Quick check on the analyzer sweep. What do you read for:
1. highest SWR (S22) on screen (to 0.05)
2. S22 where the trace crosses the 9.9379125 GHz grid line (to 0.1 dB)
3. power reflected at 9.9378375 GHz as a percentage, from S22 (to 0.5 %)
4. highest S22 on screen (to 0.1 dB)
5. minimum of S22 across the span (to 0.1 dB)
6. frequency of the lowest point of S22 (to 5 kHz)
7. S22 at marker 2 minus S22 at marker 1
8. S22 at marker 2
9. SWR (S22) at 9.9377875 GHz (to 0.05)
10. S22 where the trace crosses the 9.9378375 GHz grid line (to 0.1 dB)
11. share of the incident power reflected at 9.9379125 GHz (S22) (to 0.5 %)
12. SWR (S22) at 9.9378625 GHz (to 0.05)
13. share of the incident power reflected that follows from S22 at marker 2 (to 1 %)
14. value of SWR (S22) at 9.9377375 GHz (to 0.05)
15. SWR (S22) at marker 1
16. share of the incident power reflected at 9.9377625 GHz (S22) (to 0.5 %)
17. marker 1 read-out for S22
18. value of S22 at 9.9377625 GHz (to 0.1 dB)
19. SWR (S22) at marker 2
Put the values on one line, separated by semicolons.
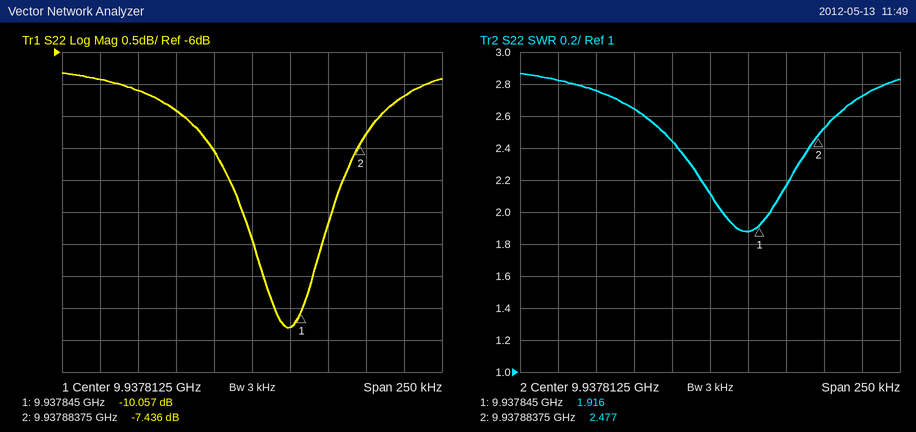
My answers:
2.85; -6.7 dB; 9.5 %; -6.3 dB; -10.3 dB; 9.937835 GHz; 2.621 dB; -7.436 dB; 2.45; -10.3 dB; 21.5 %; 2.15; 18 %; 2.75; 1.916; 20.5 %; -10.057 dB; -6.9 dB; 2.477
